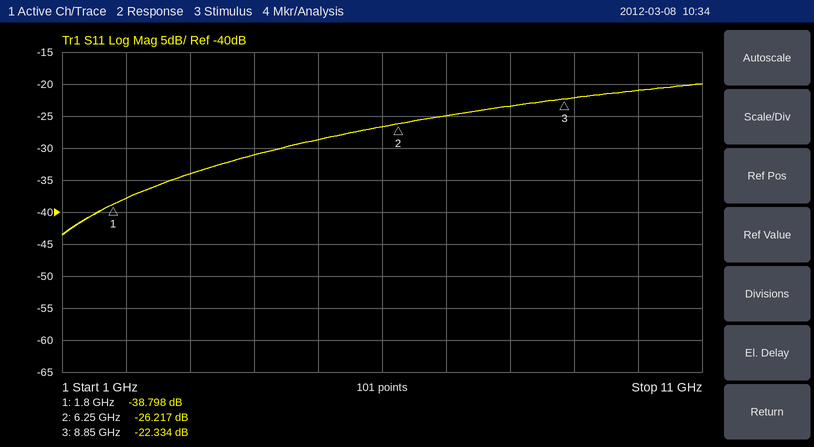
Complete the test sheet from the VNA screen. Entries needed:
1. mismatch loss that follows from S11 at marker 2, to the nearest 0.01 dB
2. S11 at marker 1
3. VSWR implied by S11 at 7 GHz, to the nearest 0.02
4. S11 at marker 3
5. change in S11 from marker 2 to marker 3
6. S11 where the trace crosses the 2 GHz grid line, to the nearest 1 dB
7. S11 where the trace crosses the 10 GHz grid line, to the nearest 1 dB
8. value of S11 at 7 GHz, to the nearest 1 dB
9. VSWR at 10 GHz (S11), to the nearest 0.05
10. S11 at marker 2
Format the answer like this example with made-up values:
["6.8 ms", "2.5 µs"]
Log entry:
["0.01 dB", "-38.798 dB", "1.12", "-22.334 dB", "3.883 dB", "-38 dB", "-21 dB", "-25 dB", "1.20", "-26.217 dB"]
